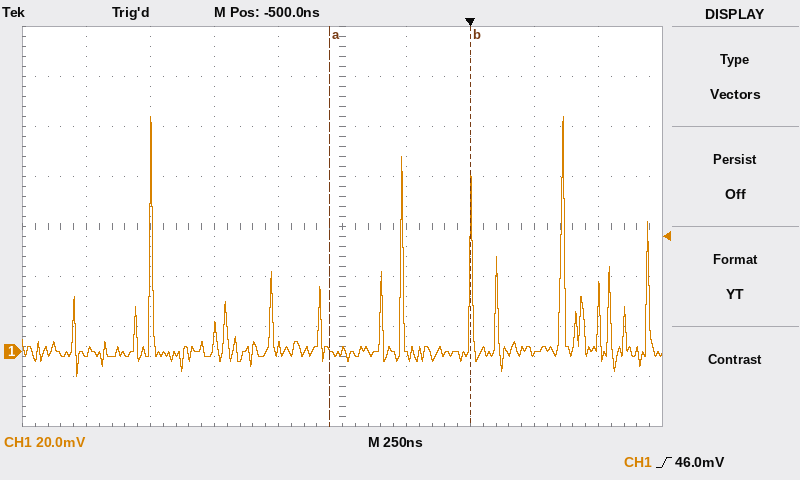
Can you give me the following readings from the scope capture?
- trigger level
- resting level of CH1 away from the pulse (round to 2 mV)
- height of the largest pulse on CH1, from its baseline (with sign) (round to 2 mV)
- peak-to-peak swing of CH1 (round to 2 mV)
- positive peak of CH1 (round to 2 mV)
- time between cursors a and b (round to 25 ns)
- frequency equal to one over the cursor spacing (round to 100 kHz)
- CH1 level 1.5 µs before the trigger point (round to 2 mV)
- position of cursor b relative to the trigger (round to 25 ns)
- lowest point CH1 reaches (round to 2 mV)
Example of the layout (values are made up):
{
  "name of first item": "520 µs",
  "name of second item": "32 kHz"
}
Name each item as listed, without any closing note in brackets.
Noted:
{
  "trigger level": "46.0 mV",
  "resting level of CH1 away from the pulse": "0 mV",
  "height of the largest pulse on CH1, from its baseline (with sign)": "+94 mV",
  "peak-to-peak swing of CH1": "104 mV",
  "positive peak of CH1": "94 mV",
  "time between cursors a and b": "550 ns",
  "frequency equal to one over the cursor spacing": "1.8 MHz",
  "CH1 level 1.5 µs before the trigger point": "0 mV",
  "position of cursor b relative to the trigger": "0 ns",
  "lowest point CH1 reaches": "-10 mV"
}
